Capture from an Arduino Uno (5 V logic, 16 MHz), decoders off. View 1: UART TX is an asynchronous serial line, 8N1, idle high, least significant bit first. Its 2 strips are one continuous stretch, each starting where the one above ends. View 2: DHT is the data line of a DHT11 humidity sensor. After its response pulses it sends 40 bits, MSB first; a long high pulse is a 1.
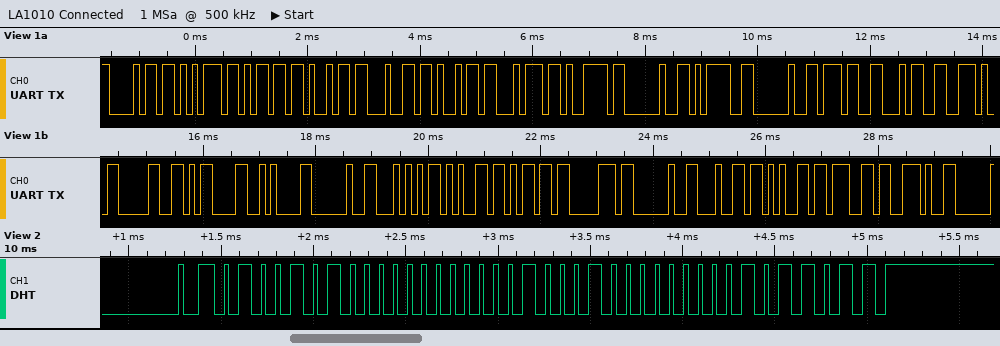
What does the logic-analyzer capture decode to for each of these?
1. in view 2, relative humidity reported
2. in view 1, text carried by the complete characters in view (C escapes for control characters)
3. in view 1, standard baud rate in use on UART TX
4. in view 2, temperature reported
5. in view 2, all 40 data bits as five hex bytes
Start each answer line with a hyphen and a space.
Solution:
- 74 %
- "humidity = 74.0\r\n Temp deg."
- 9600 baud
- 17.0 °C
- 4A 00 11 00 5B
